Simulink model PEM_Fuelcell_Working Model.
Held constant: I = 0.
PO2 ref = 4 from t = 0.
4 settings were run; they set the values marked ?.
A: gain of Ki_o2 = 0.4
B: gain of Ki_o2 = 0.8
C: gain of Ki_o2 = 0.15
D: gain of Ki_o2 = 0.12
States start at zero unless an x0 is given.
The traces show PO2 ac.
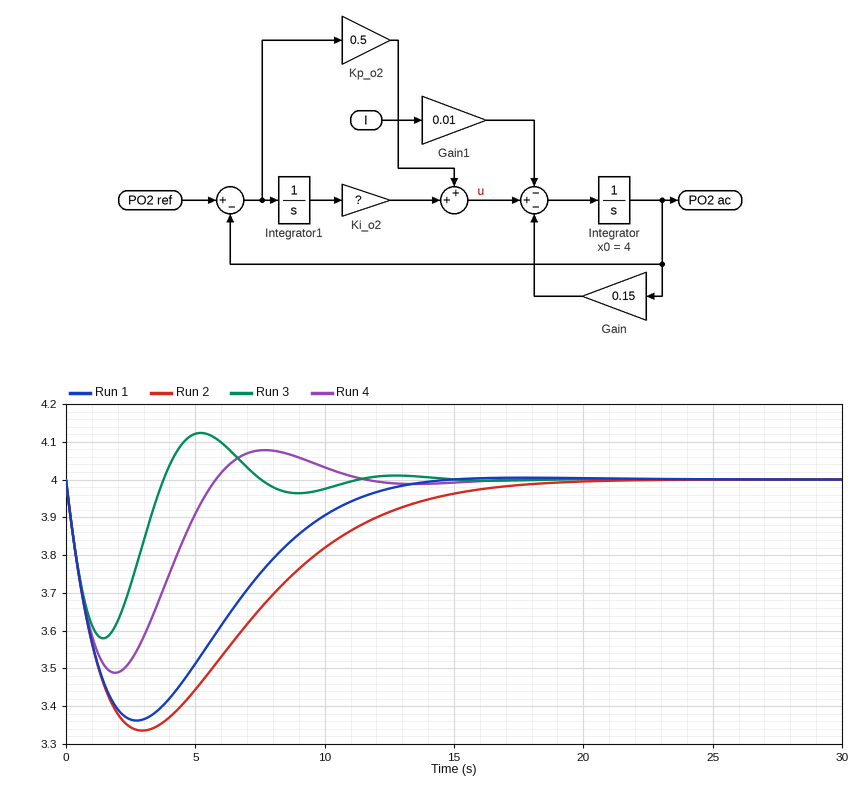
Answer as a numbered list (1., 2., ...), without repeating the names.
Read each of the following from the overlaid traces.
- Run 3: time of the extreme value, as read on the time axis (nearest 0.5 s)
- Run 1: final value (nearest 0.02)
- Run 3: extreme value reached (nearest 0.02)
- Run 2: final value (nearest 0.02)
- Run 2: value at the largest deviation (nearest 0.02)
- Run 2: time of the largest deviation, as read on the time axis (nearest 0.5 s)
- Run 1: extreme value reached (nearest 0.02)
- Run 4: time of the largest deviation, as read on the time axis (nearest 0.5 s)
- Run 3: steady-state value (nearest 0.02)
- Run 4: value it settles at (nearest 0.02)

1. 1.5 s
2. 4.00
3. 3.58
4. 4.00
5. 3.34
6. 3.0 s
7. 3.36
8. 2.0 s
9. 4.00
10. 4.00
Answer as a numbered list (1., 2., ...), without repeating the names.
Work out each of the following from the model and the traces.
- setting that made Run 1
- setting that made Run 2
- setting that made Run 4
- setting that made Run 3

1. C
2. D
3. A
4. B
